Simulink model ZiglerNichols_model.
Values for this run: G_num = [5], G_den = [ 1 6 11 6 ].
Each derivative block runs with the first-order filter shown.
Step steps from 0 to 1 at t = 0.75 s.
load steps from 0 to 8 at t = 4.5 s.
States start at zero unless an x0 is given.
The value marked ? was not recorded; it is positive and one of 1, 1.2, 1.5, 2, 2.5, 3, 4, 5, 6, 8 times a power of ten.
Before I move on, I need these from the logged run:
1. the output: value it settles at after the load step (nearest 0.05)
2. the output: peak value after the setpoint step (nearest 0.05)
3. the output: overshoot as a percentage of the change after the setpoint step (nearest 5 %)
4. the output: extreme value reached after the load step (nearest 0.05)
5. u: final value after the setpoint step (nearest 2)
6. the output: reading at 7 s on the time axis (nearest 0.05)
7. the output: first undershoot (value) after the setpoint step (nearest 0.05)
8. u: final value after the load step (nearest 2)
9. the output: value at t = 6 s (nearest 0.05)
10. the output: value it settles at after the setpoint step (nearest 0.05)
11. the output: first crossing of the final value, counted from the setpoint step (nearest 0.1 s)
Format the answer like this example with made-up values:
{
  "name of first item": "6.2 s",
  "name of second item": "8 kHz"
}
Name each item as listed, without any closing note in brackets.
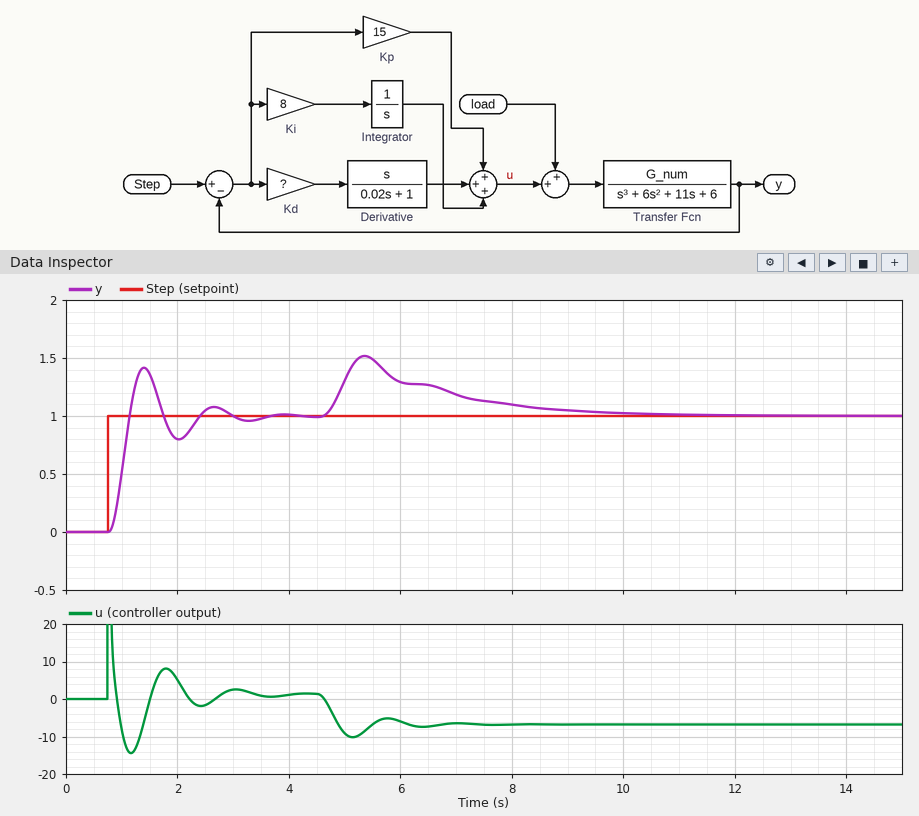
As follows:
{
  "the output: value it settles at after the load step": "1.00",
  "the output: peak value after the setpoint step": "1.40",
  "the output: overshoot as a percentage of the change after the setpoint step": "40 %",
  "the output: extreme value reached after the load step": "1.50",
  "u: final value after the setpoint step": "2",
  "the output: reading at 7 s on the time axis": "1.20",
  "the output: first undershoot (value) after the setpoint step": "0.80",
  "u: final value after the load step": "-6",
  "the output: value at t = 6 s": "1.30",
  "the output: value it settles at after the setpoint step": "1.00",
  "the output: first crossing of the final value, counted from the setpoint step": "0.4 s"
}
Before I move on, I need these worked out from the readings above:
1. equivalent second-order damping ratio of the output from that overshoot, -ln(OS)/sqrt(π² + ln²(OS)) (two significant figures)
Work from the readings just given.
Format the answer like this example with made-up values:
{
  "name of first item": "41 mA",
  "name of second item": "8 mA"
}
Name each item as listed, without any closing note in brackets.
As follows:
{
  "equivalent second-order damping ratio of the output from that overshoot, -ln(OS)/sqrt(π² + ln²(OS))": "0.28"
}
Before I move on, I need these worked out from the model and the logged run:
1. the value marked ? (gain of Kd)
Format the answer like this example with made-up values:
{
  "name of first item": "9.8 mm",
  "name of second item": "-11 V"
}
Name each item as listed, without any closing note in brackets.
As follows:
{
  "the value marked ?": "5"
}
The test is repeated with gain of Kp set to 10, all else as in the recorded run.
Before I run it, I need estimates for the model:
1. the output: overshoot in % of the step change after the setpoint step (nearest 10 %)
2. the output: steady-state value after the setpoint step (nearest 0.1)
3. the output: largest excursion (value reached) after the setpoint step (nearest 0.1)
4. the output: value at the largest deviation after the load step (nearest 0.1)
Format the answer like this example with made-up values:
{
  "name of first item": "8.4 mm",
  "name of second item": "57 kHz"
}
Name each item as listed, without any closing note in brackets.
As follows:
{
  "the output: overshoot in % of the step change after the setpoint step": "30 %",
  "the output: steady-state value after the setpoint step": "1.0",
  "the output: largest excursion (value reached) after the setpoint step": "1.3",
  "the output: value at the largest deviation after the load step": "1.6"
}
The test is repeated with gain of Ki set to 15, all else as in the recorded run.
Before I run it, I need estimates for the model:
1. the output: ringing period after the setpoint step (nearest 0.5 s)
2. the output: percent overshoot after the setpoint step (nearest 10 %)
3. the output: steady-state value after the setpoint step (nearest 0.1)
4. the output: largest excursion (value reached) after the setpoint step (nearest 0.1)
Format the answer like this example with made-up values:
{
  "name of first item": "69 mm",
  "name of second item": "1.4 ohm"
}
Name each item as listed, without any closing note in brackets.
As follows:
{
  "the output: ringing period after the setpoint step": "1.5 s",
  "the output: percent overshoot after the setpoint step": "50 %",
  "the output: steady-state value after the setpoint step": "1.0",
  "the output: largest excursion (value reached) after the setpoint step": "1.5"
}
